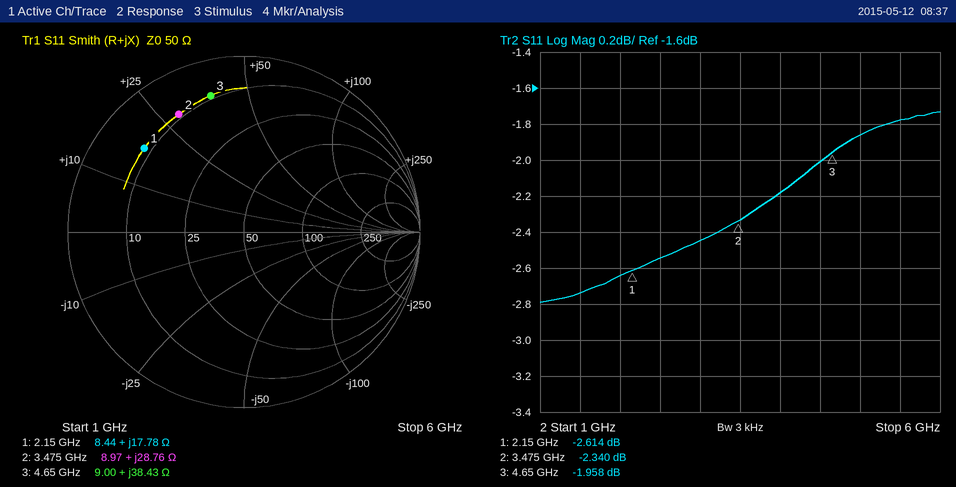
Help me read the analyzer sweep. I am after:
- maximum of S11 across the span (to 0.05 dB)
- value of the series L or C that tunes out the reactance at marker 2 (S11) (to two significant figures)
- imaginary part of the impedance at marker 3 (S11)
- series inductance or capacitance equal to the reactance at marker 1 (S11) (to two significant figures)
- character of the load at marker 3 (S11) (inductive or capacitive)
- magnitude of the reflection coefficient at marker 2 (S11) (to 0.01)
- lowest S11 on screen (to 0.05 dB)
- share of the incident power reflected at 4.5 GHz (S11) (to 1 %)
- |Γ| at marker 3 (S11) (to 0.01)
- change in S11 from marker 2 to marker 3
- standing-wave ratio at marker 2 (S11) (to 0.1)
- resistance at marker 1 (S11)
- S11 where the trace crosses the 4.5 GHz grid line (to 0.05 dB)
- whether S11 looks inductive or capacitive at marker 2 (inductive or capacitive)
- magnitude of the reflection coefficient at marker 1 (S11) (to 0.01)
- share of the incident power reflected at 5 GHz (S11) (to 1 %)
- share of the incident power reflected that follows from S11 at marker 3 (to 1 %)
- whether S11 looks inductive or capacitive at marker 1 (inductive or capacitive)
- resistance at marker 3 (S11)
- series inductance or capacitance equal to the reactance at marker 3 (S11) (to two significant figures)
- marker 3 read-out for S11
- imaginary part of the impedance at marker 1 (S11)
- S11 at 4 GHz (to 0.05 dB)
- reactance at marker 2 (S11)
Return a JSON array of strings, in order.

["-1.75 dB", "1.6 pF", "+38.43 Ω", "1.3 nH", "inductive", "0.76", "-2.80 dB", "63 %", "0.80", "0.382 dB", "7.5", "8.44 Ω", "-2.00 dB", "inductive", "0.74", "65 %", "64 %", "inductive", "9.00 Ω", "1.3 nH", "-1.958 dB", "+17.78 Ω", "-2.20 dB", "+28.76 Ω"]
